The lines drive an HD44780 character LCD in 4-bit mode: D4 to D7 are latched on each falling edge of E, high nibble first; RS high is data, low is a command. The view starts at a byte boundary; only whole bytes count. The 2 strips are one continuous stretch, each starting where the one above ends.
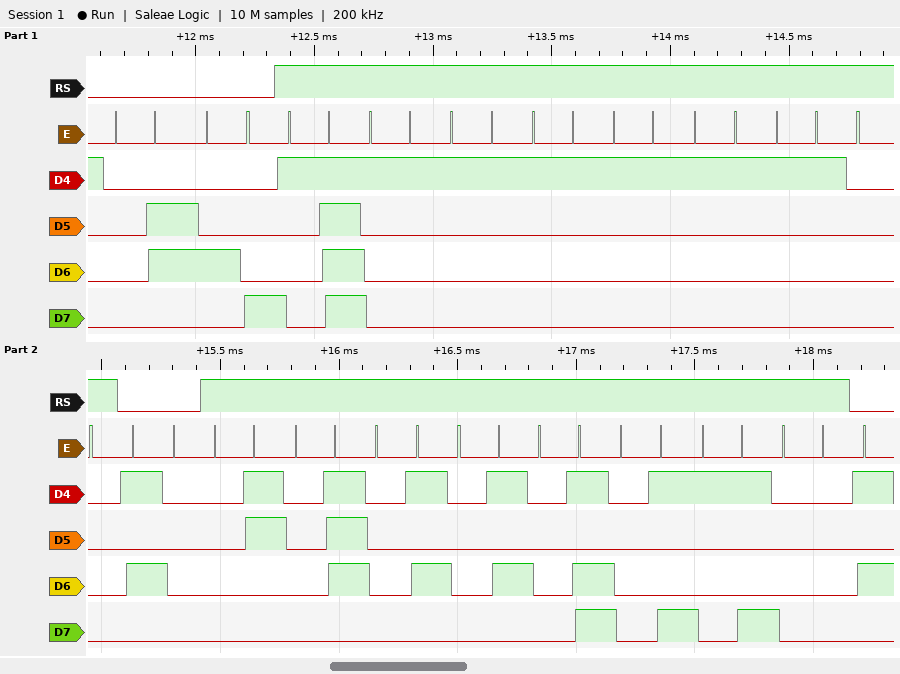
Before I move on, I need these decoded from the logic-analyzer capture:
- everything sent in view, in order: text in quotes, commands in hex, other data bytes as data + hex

0x06 0x48 data 1F 11 11 11 11 11 11 00 0x50 data 03 07 05 05 0D 09 19 00
